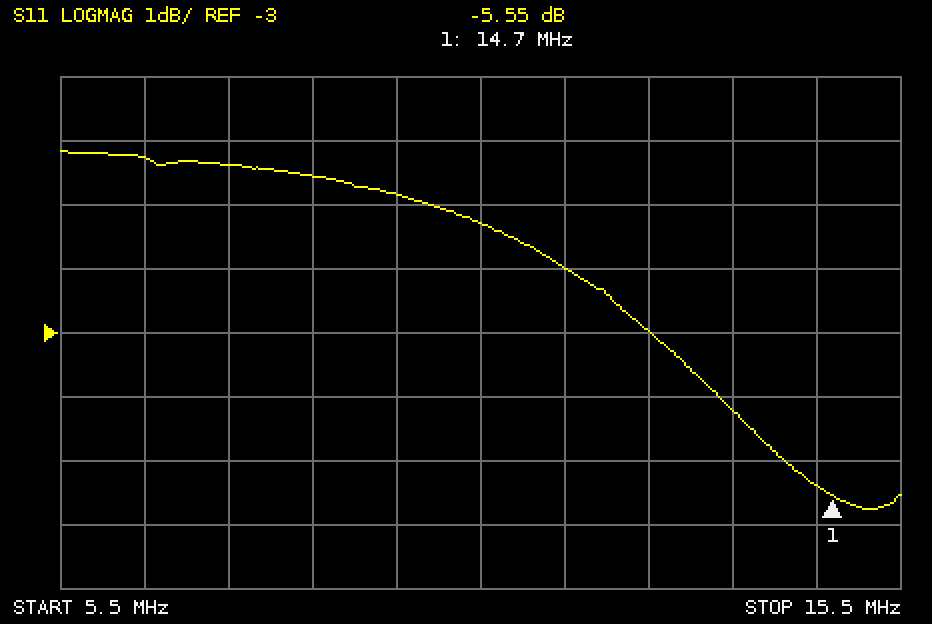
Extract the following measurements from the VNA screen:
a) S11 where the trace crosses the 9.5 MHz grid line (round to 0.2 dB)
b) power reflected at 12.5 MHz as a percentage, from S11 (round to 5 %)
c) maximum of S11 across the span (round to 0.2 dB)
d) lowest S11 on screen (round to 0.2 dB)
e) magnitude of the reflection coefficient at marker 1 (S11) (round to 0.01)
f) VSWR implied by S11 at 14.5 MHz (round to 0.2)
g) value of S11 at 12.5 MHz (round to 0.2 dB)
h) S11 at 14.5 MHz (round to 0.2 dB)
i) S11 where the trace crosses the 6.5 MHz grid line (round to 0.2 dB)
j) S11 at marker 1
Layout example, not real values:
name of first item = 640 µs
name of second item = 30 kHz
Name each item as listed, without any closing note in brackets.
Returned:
S11 where the trace crosses the 9.5 MHz grid line = -0.8 dB
power reflected at 12.5 MHz as a percentage, from S11 = 50 %
maximum of S11 across the span = -0.2 dB
lowest S11 on screen = -5.8 dB
magnitude of the reflection coefficient at marker 1 (S11) = 0.53
VSWR implied by S11 at 14.5 MHz = 3.4
value of S11 at 12.5 MHz = -3.0 dB
S11 at 14.5 MHz = -5.4 dB
S11 where the trace crosses the 6.5 MHz grid line = -0.2 dB
S11 at marker 1 = -5.55 dB
